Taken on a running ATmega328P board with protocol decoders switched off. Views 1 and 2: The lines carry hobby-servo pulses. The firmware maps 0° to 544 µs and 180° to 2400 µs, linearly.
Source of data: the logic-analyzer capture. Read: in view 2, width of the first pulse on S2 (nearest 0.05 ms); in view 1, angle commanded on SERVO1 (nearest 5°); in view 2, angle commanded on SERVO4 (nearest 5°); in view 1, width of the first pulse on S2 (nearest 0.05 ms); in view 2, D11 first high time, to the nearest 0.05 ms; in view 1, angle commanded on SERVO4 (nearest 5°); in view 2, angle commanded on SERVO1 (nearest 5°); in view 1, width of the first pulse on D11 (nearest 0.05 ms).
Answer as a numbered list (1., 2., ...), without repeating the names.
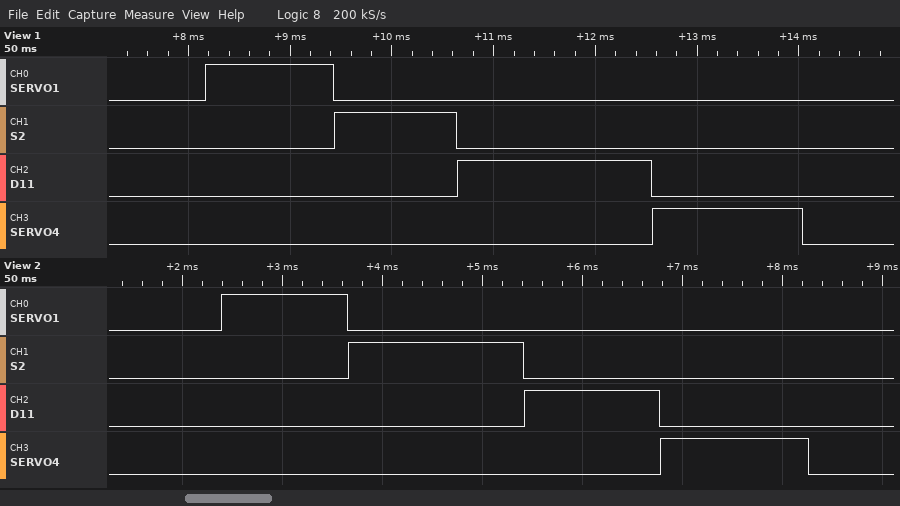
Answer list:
1. 1.75 ms
2. 70°
3. 90°
4. 1.20 ms
5. 1.35 ms
6. 90°
7. 70°
8. 1.90 ms
